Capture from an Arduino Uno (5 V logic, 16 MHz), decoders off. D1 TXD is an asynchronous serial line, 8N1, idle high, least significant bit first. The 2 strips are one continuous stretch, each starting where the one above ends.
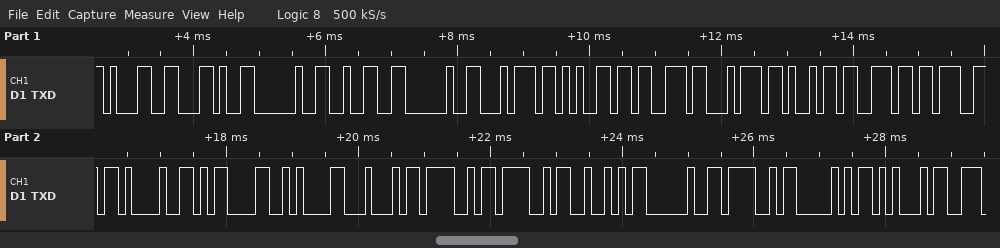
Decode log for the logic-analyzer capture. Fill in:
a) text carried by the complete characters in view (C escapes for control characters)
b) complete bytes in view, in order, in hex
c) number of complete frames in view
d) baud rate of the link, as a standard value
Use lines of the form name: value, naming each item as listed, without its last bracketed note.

text carried by the complete characters in view: "1, 2 testing!\r\nDOOR OPE"
complete bytes in view, in order, in hex: 31 2C 20 32 20 74 65 73 74 69 6E 67 21 0D 0A 44 4F 4F 52 20 4F 50 45
number of complete frames in view: 23
baud rate of the link, as a standard value: 9600 baud
